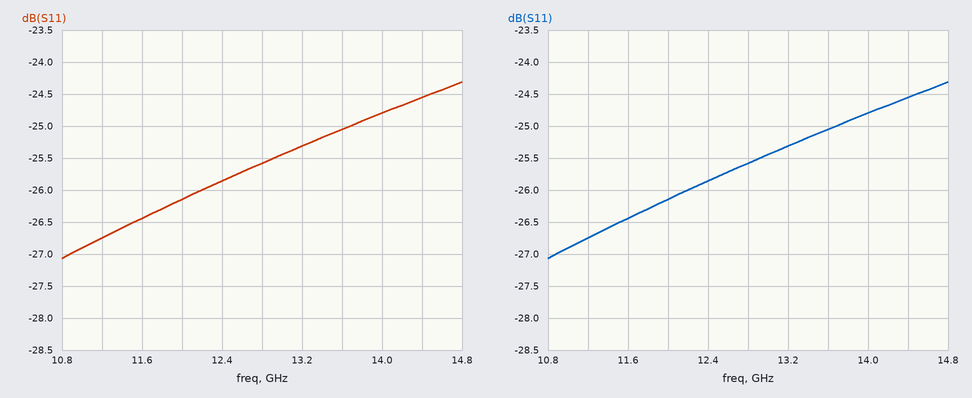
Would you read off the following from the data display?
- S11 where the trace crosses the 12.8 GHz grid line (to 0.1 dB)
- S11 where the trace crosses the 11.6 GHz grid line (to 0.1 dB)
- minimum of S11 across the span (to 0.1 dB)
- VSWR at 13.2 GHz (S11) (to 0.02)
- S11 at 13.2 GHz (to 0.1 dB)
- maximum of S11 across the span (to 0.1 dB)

-25.6 dB
-26.4 dB
-27.1 dB
1.12
-25.3 dB
-24.3 dB
